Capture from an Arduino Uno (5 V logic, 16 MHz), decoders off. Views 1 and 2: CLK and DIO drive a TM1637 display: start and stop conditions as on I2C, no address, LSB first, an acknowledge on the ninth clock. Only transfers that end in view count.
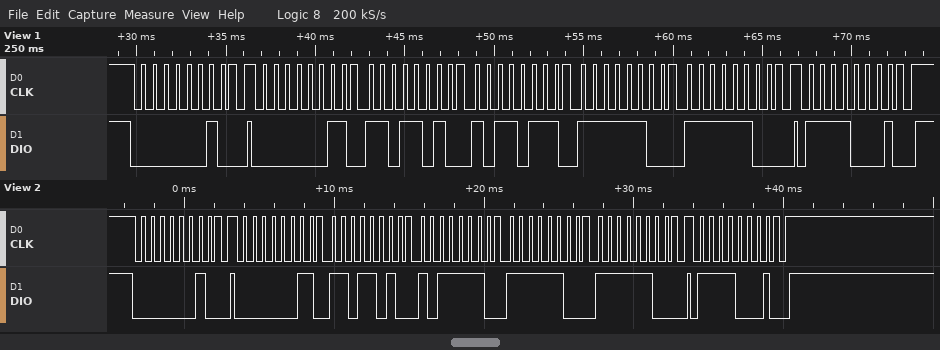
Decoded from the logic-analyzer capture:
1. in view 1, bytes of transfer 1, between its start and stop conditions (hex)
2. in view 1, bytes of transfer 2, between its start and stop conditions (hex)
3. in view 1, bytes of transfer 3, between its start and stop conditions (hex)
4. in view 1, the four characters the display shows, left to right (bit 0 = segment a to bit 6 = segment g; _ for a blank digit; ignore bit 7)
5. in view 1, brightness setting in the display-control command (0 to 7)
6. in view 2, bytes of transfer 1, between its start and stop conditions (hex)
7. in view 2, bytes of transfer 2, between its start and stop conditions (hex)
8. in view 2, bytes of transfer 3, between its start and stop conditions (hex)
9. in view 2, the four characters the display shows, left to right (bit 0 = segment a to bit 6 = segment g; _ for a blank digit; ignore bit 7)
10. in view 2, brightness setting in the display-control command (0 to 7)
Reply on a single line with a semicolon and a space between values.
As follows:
40; C0 5B ED 3F 3F; 8F; 2500; 7; 40; C0 5B 7D 3F 3F; 8F; 2600; 7
